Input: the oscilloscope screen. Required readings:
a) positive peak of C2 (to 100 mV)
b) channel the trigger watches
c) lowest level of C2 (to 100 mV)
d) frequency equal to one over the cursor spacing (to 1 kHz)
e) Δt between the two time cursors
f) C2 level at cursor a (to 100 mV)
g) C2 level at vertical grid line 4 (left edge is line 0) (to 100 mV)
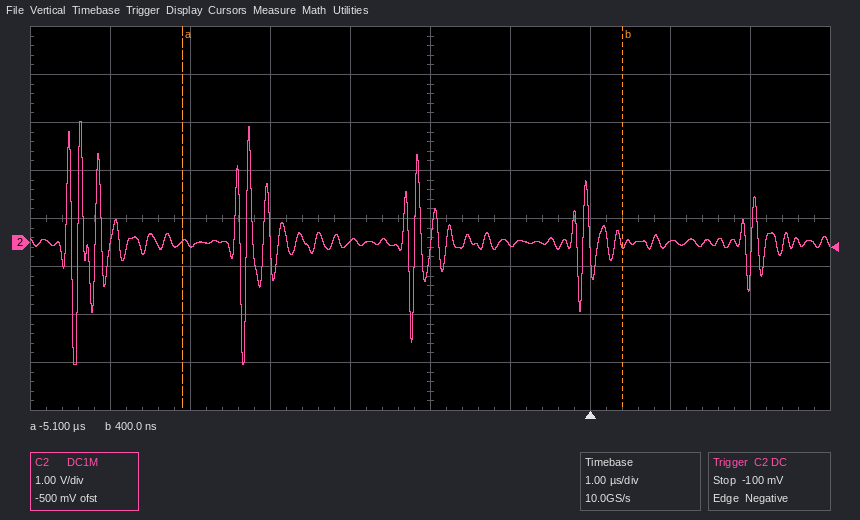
2.5 V
C2
-2.5 V
182 kHz
5.5 µs
0.0 V
0.0 V
